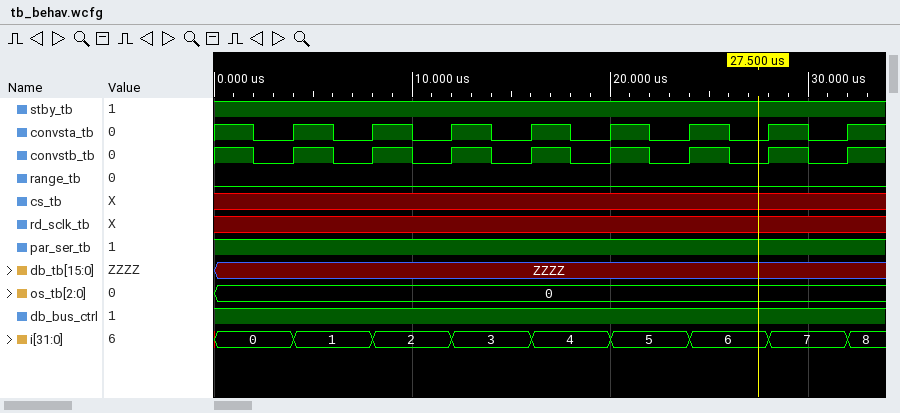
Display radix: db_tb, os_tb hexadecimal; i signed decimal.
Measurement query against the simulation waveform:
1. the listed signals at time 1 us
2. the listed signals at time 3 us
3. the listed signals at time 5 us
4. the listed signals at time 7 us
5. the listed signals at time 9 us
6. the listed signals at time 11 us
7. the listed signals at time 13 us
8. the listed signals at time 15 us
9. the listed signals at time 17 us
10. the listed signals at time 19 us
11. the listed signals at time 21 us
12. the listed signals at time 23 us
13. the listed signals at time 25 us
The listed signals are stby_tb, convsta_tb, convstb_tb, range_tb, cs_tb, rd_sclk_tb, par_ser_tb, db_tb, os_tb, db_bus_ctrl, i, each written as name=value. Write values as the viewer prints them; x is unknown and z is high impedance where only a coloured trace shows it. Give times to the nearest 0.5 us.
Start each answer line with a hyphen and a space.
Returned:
- stby_tb=1, convsta_tb=1, convstb_tb=1, range_tb=0, cs_tb=x, rd_sclk_tb=x, par_ser_tb=1, db_tb=ZZZZ, os_tb=0, db_bus_ctrl=1, i=0
- stby_tb=1, convsta_tb=0, convstb_tb=0, range_tb=0, cs_tb=x, rd_sclk_tb=x, par_ser_tb=1, db_tb=ZZZZ, os_tb=0, db_bus_ctrl=1, i=0
- stby_tb=1, convsta_tb=1, convstb_tb=1, range_tb=0, cs_tb=x, rd_sclk_tb=x, par_ser_tb=1, db_tb=ZZZZ, os_tb=0, db_bus_ctrl=1, i=1
- stby_tb=1, convsta_tb=0, convstb_tb=0, range_tb=0, cs_tb=x, rd_sclk_tb=x, par_ser_tb=1, db_tb=ZZZZ, os_tb=0, db_bus_ctrl=1, i=1
- stby_tb=1, convsta_tb=1, convstb_tb=1, range_tb=0, cs_tb=x, rd_sclk_tb=x, par_ser_tb=1, db_tb=ZZZZ, os_tb=0, db_bus_ctrl=1, i=2
- stby_tb=1, convsta_tb=0, convstb_tb=0, range_tb=0, cs_tb=x, rd_sclk_tb=x, par_ser_tb=1, db_tb=ZZZZ, os_tb=0, db_bus_ctrl=1, i=2
- stby_tb=1, convsta_tb=1, convstb_tb=1, range_tb=0, cs_tb=x, rd_sclk_tb=x, par_ser_tb=1, db_tb=ZZZZ, os_tb=0, db_bus_ctrl=1, i=3
- stby_tb=1, convsta_tb=0, convstb_tb=0, range_tb=0, cs_tb=x, rd_sclk_tb=x, par_ser_tb=1, db_tb=ZZZZ, os_tb=0, db_bus_ctrl=1, i=3
- stby_tb=1, convsta_tb=1, convstb_tb=1, range_tb=0, cs_tb=x, rd_sclk_tb=x, par_ser_tb=1, db_tb=ZZZZ, os_tb=0, db_bus_ctrl=1, i=4
- stby_tb=1, convsta_tb=0, convstb_tb=0, range_tb=0, cs_tb=x, rd_sclk_tb=x, par_ser_tb=1, db_tb=ZZZZ, os_tb=0, db_bus_ctrl=1, i=4
- stby_tb=1, convsta_tb=1, convstb_tb=1, range_tb=0, cs_tb=x, rd_sclk_tb=x, par_ser_tb=1, db_tb=ZZZZ, os_tb=0, db_bus_ctrl=1, i=5
- stby_tb=1, convsta_tb=0, convstb_tb=0, range_tb=0, cs_tb=x, rd_sclk_tb=x, par_ser_tb=1, db_tb=ZZZZ, os_tb=0, db_bus_ctrl=1, i=5
- stby_tb=1, convsta_tb=1, convstb_tb=1, range_tb=0, cs_tb=x, rd_sclk_tb=x, par_ser_tb=1, db_tb=ZZZZ, os_tb=0, db_bus_ctrl=1, i=6
